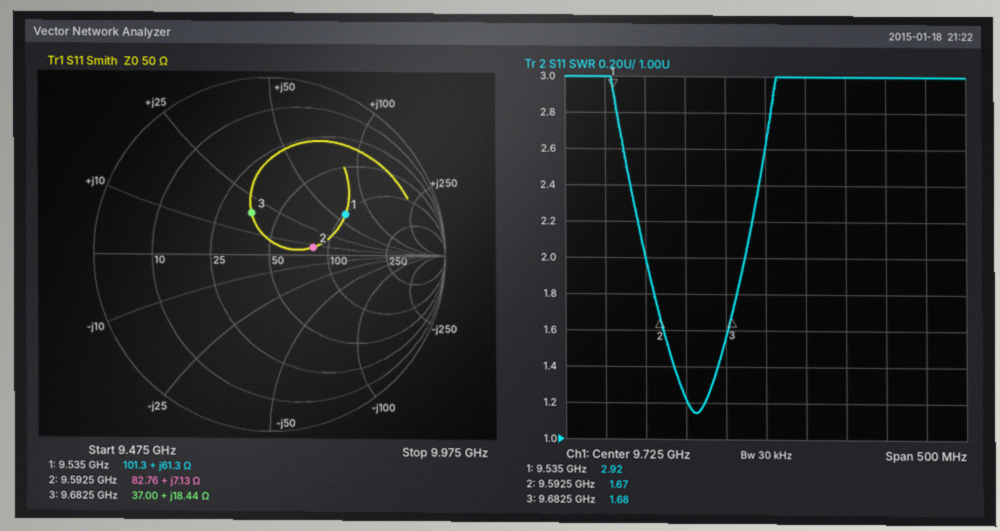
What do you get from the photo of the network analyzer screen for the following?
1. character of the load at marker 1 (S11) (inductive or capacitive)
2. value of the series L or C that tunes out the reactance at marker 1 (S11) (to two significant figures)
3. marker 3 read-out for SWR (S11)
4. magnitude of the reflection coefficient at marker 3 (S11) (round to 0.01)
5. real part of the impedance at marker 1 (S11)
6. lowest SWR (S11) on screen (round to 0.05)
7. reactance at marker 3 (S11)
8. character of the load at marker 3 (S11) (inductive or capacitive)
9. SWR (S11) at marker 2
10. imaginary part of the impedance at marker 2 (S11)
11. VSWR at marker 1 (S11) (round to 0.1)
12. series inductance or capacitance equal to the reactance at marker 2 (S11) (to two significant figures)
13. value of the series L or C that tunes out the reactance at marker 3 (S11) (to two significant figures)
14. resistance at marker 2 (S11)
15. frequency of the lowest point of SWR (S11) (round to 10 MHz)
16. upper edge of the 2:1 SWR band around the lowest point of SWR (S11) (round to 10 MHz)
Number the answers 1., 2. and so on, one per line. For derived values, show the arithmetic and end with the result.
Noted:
1. inductive
2. C = 1/(2π × 9.535 GHz × 61.3 Ω) ≈ 272 fF, so 270 fF to two significant figures
3. 1.68
4. 0.25
5. 101.3 Ω
6. 1.15
7. +18.44 Ω
8. inductive
9. 1.67
10. +7.13 Ω
11. 2.9
12. L = 7.13 Ω/(2π × 9.5925 GHz) ≈ 118 pH, so 120 pH to two significant figures
13. C = 1/(2π × 9.6825 GHz × 18.44 Ω) ≈ 891 fF, so 890 fF to two significant figures
14. 82.76 Ω
15. 9.64 GHz
16. 9.70 GHz
